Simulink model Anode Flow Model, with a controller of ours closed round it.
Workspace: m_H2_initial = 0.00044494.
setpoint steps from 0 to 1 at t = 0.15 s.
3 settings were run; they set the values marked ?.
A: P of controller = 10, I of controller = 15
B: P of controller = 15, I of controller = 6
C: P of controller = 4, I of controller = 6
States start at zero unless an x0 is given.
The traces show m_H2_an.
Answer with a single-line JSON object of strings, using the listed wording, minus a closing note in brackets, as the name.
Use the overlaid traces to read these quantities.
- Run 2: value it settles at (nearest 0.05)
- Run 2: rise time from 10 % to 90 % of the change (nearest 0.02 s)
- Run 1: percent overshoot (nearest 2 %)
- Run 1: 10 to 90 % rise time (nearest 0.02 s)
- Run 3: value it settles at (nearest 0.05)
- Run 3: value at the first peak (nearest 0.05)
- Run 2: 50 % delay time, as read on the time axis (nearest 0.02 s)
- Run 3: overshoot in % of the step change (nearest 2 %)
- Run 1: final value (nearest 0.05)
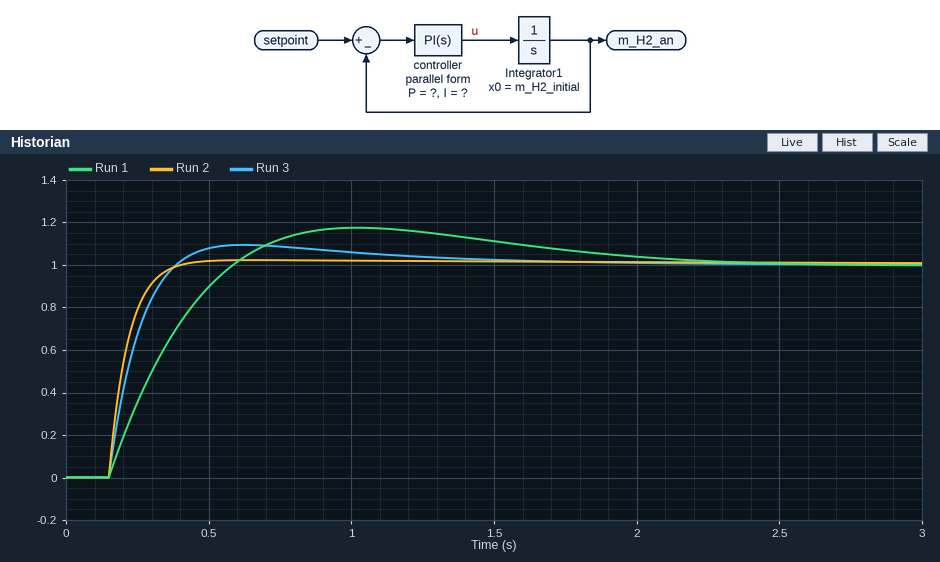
{"Run 2: value it settles at": "1.00", "Run 2: rise time from 10 % to 90 % of the change": "0.14 s", "Run 1: percent overshoot": "18 %", "Run 1: 10 to 90 % rise time": "0.32 s", "Run 3: value it settles at": "1.00", "Run 3: value at the first peak": "1.10", "Run 2: 50 % delay time, as read on the time axis": "0.20 s", "Run 3: overshoot in % of the step change": "10 %", "Run 1: final value": "1.00"}
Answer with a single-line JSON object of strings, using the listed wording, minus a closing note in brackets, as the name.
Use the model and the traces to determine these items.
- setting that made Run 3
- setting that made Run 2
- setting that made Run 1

{"setting that made Run 3": "A", "setting that made Run 2": "B", "setting that made Run 1": "C"}
